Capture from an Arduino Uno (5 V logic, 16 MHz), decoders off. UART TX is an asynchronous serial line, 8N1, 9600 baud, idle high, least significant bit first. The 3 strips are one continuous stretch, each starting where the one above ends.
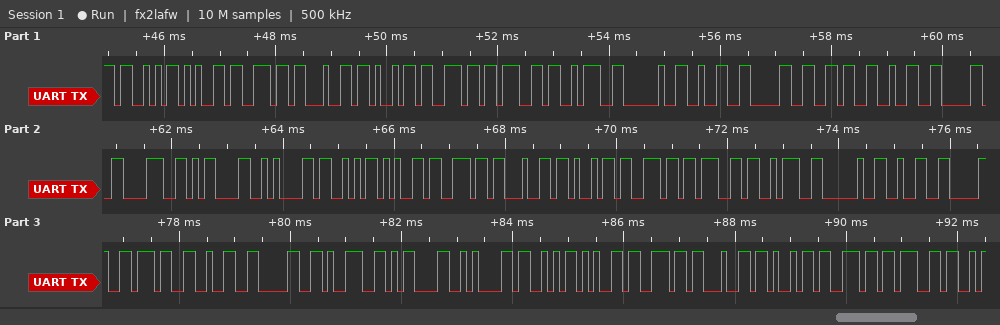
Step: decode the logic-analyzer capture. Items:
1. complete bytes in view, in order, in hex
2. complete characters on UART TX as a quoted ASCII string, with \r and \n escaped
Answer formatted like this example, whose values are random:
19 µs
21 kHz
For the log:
53 65 6E 64 69 6E 67 3A 20 32 30 36 32 30 38 0D 0A 53 65 6E 64 69 6E 67 3A 20 32 30 37 32 30 39 0D 0A 53 65 6E 64 69 6E 67
"Sending: 206208\r\nSending: 207209\r\nSending"
